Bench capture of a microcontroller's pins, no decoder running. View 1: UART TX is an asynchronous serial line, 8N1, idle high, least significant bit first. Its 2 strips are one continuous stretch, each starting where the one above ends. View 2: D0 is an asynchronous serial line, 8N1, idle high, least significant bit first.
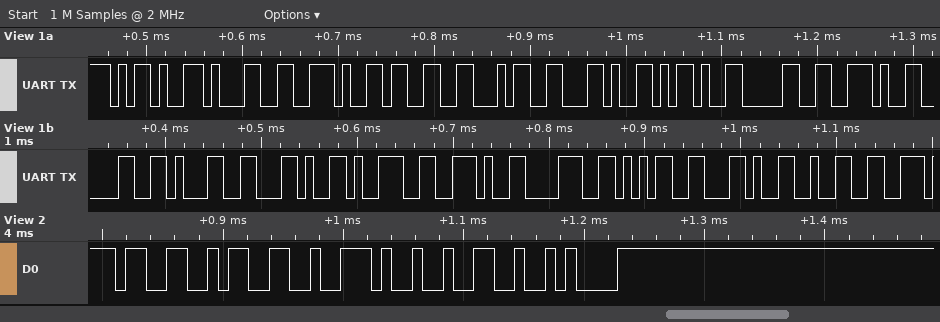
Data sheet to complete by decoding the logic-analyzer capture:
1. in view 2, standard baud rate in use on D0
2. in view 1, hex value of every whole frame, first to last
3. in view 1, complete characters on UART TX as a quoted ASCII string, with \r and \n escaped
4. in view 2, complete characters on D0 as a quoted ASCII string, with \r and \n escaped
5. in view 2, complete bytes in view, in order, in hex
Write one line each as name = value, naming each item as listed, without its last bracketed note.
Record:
in view 2, standard baud rate in use on D0 = 115200 baud
in view 1, hex value of every whole frame, first to last = 2D 31 2E 33 34 2C 2D 30 2E 30 31 2C 39 2E 38 35 2C 32
in view 1, complete characters on UART TX as a quoted ASCII string, with \r and \n escaped = "-1.34,-0.01,9.85,2"
in view 2, complete characters on D0 as a quoted ASCII string, with \r and \n escaped = "33.2\n"
in view 2, complete bytes in view, in order, in hex = 33 33 2E 32 0A
